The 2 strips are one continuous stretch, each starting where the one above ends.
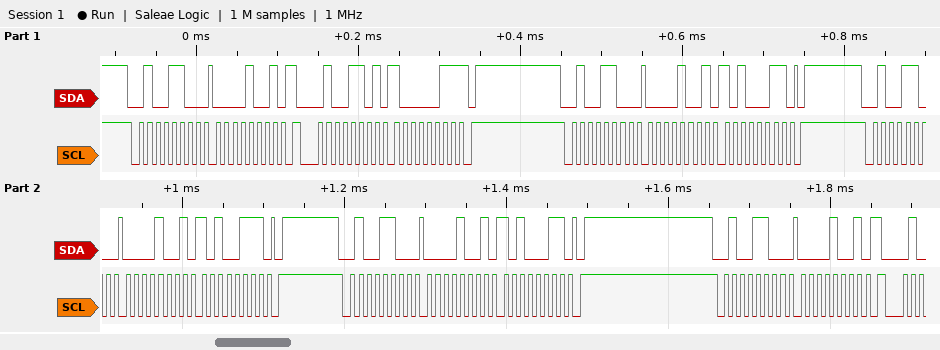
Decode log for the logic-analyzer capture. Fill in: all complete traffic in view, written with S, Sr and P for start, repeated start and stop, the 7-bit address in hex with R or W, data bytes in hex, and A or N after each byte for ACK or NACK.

S 26W A 09 A Sr 26R A 83 N P S 26W A 09 A A3 A P S 26W A 09 A A7 A P S 26W A 09 A A3 A P S 26W A 09 A
